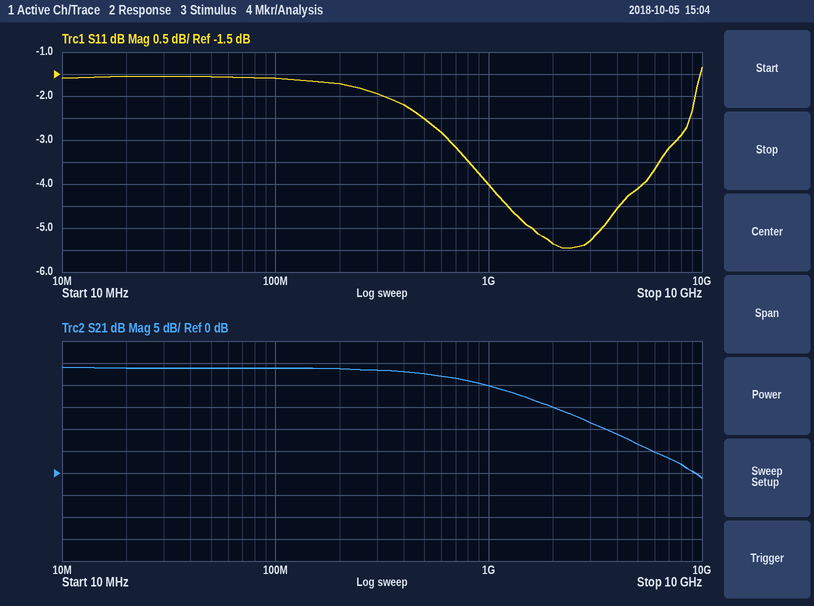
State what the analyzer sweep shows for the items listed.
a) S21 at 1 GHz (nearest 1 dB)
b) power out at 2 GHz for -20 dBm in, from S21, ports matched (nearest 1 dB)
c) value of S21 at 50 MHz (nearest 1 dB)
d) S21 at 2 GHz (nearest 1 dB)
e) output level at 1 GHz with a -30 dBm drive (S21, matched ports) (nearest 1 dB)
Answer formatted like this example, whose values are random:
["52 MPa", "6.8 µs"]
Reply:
["20 dB", "-5 dBm", "24 dB", "15 dB", "-10 dBm"]
